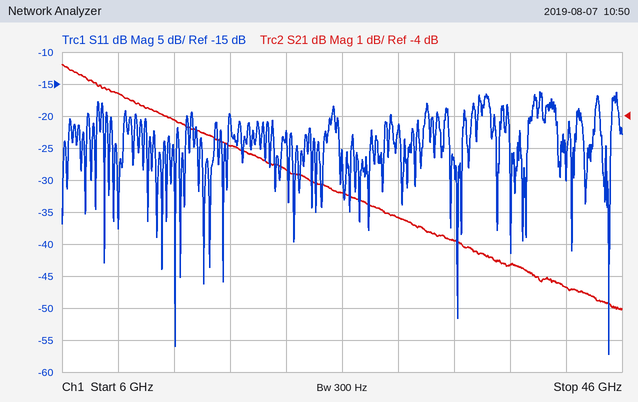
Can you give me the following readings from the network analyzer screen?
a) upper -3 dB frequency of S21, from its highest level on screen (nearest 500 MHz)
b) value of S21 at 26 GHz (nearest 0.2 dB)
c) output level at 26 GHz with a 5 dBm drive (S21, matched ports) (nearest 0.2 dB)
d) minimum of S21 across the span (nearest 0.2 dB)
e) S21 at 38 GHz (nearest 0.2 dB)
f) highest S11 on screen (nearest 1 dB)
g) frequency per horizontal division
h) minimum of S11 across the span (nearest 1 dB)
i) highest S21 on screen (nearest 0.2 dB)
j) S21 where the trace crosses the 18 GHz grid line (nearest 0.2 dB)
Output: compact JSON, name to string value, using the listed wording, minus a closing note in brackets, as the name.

{"upper -3 dB frequency of S21, from its highest level on screen": "20.5 GHz", "value of S21 at 26 GHz": "-6.4 dB", "output level at 26 GHz with a 5 dBm drive (S21, matched ports)": "-1.4 dBm", "minimum of S21 across the span": "-10.0 dB", "S21 at 38 GHz": "-8.6 dB", "highest S11 on screen": "-16 dB", "frequency per horizontal division": "4 GHz", "minimum of S11 across the span": "-57 dB", "highest S21 on screen": "-2.4 dB", "S21 where the trace crosses the 18 GHz grid line": "-5.0 dB"}
